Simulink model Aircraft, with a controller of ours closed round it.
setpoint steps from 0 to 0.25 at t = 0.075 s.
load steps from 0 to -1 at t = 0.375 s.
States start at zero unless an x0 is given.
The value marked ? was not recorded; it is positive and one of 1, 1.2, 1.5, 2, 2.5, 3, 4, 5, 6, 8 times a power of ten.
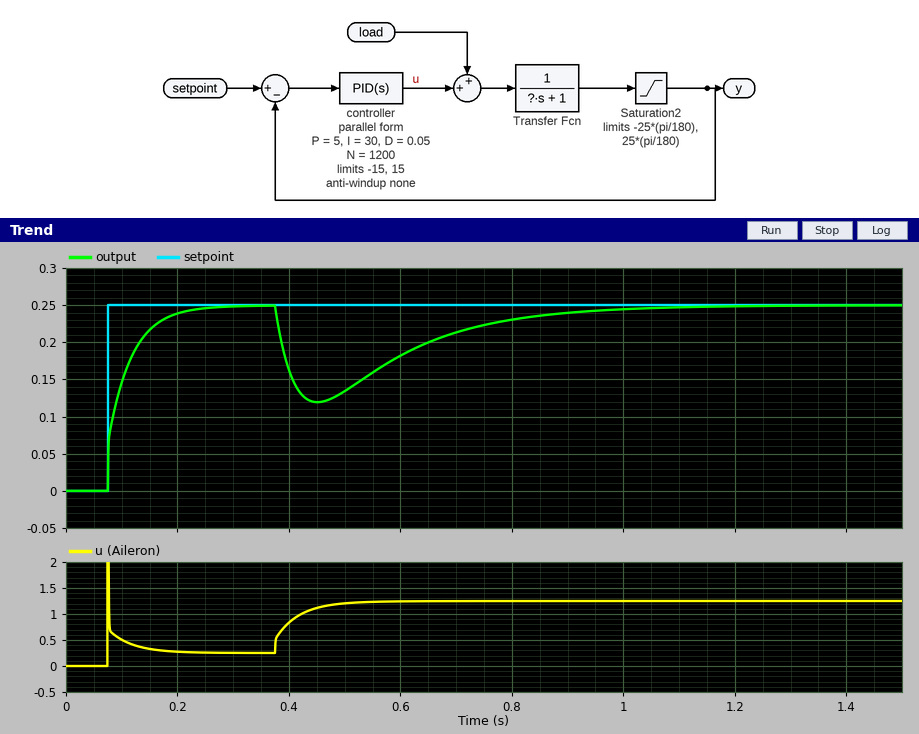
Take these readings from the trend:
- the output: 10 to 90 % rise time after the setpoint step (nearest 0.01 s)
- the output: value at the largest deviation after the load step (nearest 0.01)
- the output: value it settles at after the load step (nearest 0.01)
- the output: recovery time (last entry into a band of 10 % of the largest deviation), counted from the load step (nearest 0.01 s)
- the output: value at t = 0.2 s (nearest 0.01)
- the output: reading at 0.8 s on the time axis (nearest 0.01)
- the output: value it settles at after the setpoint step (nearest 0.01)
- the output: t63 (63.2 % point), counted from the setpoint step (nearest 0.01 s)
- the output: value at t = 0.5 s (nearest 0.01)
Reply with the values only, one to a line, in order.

0.09 s
0.12
0.25
0.49 s
0.24
0.23
0.25
0.03 s
0.13
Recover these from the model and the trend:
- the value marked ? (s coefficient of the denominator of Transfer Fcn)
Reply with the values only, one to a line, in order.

0.15
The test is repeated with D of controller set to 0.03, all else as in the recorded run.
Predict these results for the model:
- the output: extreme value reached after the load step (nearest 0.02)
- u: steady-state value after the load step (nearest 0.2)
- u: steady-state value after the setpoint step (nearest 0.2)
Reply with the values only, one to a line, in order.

0.12
1.2
0.2
